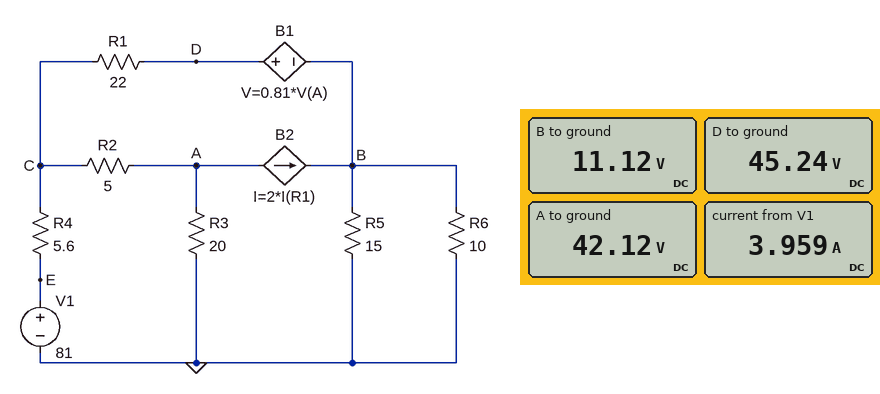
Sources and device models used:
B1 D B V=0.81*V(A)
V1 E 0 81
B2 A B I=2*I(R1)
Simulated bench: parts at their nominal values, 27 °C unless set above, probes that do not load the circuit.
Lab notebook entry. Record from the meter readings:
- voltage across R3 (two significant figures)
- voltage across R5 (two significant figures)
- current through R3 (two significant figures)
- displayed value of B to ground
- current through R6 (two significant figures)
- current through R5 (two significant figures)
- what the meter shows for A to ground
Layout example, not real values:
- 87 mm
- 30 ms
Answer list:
- 42 V
- 11 V
- 2.1 A
- 11.12 V
- 1.1 A
- 740 mA
- 42.12 V
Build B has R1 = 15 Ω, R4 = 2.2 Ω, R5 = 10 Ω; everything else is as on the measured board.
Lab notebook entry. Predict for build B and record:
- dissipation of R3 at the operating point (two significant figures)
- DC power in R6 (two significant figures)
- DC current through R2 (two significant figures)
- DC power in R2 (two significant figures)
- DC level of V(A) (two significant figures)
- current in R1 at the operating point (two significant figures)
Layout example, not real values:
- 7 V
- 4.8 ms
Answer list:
- 110 W
- 24 W
- 4.4 A
- 97 W
- 47 V
- 1.0 A
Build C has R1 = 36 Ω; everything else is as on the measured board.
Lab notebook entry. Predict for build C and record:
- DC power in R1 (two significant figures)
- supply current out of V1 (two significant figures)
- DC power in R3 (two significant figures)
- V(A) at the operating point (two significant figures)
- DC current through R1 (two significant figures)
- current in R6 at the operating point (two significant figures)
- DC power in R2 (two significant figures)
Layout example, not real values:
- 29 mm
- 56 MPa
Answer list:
- 7.3 W
- 3.6 A
- 100 W
- 45 V
- 450 mA
- 810 mA
- 50 W
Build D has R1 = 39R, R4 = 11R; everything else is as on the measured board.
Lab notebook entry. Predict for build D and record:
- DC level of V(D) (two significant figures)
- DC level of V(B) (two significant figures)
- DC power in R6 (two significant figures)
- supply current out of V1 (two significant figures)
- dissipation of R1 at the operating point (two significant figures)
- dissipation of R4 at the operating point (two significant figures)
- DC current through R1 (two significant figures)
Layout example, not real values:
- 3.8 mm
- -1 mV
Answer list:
- 36 V
- 6.2 V
- 3.8 W
- 2.9 A
- 4.6 W
- 91 W
- 340 mA
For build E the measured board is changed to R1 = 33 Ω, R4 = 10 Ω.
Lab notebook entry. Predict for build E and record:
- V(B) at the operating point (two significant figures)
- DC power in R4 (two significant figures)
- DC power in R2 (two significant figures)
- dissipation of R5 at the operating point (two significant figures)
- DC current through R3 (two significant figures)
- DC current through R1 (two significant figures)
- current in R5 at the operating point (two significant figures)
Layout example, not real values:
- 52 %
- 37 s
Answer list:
- 7.2 V
- 93 W
- 35 W
- 3.4 W
- 1.9 A
- 400 mA
- 480 mA
